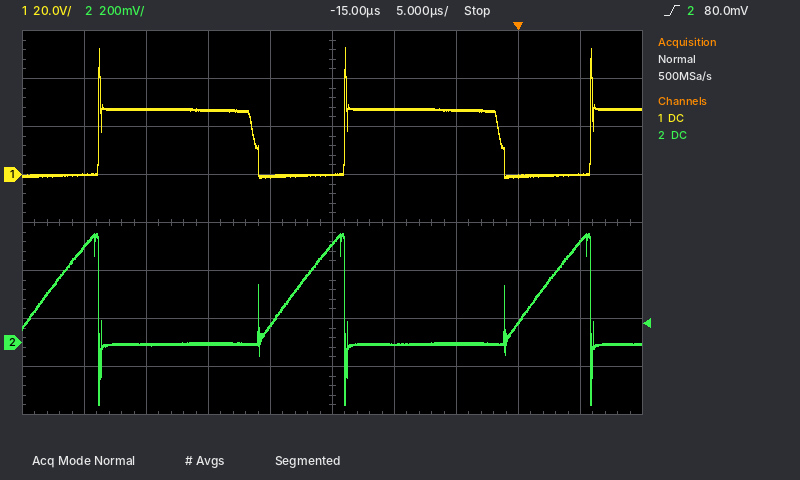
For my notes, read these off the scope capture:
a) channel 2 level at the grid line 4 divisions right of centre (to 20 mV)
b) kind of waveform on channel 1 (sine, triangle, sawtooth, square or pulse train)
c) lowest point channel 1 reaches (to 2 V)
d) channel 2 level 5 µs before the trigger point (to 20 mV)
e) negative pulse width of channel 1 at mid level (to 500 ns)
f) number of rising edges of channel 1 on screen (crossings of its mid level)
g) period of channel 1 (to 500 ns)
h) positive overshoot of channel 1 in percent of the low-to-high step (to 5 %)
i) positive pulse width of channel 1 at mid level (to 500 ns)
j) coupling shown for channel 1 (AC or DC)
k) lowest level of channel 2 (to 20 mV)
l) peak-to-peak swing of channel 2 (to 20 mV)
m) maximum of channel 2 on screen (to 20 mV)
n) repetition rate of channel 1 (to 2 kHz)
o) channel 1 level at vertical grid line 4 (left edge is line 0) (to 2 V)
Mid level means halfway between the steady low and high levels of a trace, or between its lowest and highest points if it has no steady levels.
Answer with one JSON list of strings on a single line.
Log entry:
["420 mV", "pulse train", "-2 V", "0 mV", "7.0 µs", "3", "20.0 µs", "95 %", "12.5 µs", "DC", "-260 mV", "720 mV", "460 mV", "50 kHz", "0 V"]
